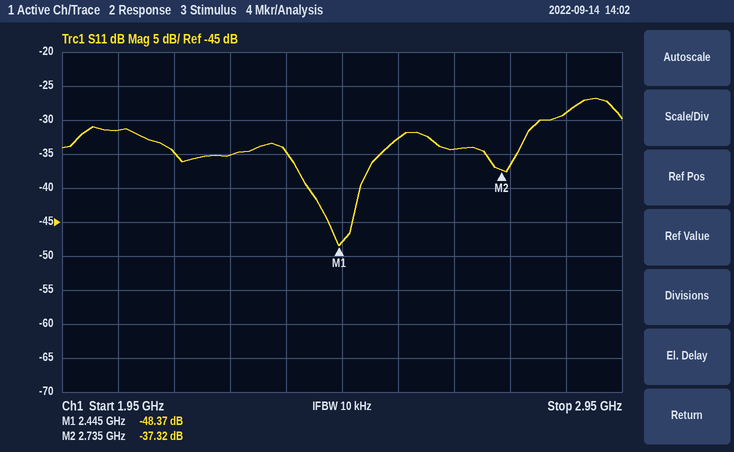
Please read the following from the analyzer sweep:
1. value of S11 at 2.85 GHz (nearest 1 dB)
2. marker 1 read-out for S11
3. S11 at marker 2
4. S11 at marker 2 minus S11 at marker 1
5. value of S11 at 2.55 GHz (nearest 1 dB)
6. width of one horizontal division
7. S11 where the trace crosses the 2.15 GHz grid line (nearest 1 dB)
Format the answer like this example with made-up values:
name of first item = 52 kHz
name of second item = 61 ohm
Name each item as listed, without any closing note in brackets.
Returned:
value of S11 at 2.85 GHz = -29 dB
marker 1 read-out for S11 = -48.37 dB
S11 at marker 2 = -37.32 dB
S11 at marker 2 minus S11 at marker 1 = 11.05 dB
value of S11 at 2.55 GHz = -33 dB
width of one horizontal division = 100 MHz
S11 where the trace crosses the 2.15 GHz grid line = -35 dB
